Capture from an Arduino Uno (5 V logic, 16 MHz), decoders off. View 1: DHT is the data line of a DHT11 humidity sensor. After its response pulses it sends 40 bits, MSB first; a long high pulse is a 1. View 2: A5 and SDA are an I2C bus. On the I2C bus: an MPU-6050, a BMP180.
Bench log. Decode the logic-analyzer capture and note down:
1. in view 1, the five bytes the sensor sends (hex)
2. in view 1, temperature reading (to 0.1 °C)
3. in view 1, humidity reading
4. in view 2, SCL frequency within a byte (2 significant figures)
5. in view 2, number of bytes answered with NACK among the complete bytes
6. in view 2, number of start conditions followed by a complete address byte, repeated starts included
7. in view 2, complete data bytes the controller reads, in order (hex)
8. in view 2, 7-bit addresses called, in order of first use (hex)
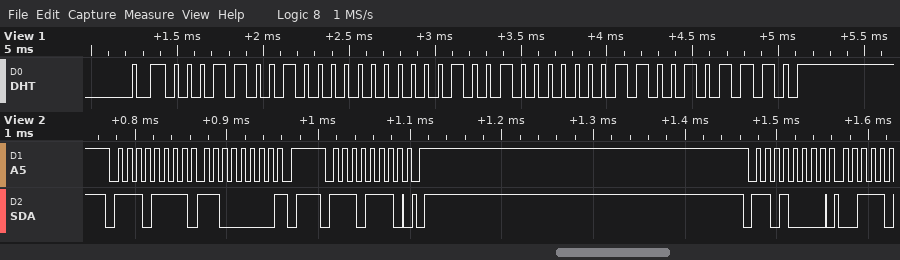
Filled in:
19 00 12 03 2E
18.3 °C
25 %
100 kHz
1
3
C0
0x77 0x68
